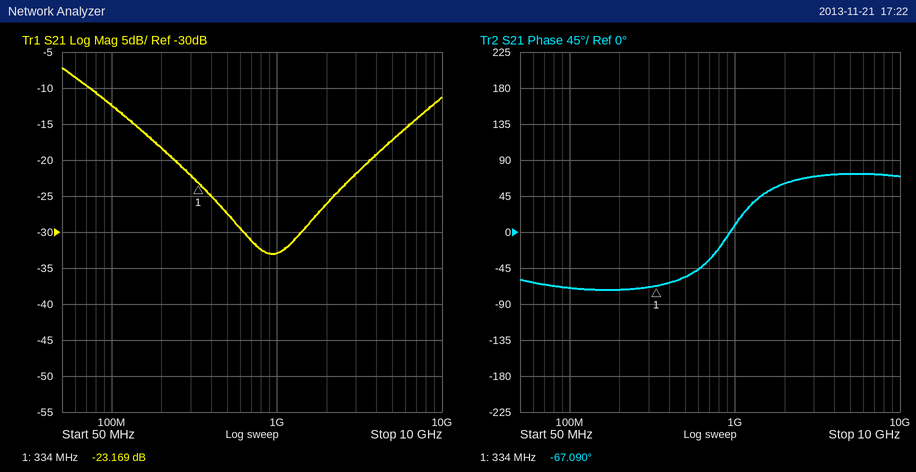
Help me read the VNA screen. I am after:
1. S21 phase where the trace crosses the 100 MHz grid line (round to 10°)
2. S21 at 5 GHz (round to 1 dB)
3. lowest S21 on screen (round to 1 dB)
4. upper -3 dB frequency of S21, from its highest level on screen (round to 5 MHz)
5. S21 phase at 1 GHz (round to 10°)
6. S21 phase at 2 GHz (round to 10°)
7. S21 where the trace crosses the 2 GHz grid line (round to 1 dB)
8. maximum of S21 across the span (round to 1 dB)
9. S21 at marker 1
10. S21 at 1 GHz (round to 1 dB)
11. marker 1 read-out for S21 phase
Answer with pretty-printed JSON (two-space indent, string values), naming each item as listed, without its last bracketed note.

{
  "S21 phase where the trace crosses the 100 MHz grid line": "-70°",
  "S21 at 5 GHz": "-17 dB",
  "lowest S21 on screen": "-33 dB",
  "upper -3 dB frequency of S21, from its highest level on screen": "75 MHz",
  "S21 phase at 1 GHz": "10°",
  "S21 phase at 2 GHz": "60°",
  "S21 where the trace crosses the 2 GHz grid line": "-26 dB",
  "maximum of S21 across the span": "-7 dB",
  "S21 at marker 1": "-23.169 dB",
  "S21 at 1 GHz": "-33 dB",
  "marker 1 read-out for S21 phase": "-67.090°"
}
